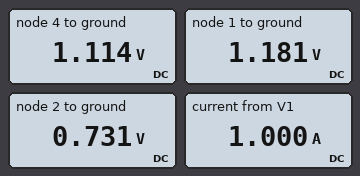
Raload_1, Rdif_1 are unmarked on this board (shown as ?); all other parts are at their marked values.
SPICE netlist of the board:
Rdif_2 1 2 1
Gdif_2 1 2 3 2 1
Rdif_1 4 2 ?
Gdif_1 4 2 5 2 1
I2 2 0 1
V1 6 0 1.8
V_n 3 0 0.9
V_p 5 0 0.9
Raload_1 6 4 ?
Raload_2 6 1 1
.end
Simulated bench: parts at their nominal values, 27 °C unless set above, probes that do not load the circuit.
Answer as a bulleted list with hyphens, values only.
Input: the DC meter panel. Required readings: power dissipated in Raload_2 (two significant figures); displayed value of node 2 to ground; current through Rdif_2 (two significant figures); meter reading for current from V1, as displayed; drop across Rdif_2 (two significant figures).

- 380 mW
- 0.731 V
- 450 mA
- 1.000 A
- 450 mV
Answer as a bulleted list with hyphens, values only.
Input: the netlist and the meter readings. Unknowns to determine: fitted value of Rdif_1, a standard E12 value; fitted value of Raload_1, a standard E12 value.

- 1.8 Ω
- 1.8 Ω
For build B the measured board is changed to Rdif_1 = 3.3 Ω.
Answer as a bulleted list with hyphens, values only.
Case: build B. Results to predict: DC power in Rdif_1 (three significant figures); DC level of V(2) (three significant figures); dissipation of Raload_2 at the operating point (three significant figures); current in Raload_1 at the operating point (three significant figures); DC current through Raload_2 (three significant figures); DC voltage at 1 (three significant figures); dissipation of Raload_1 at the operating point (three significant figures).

- 69.1 mW
- 697 mV
- 426 mW
- 347 mA
- 653 mA
- 1.15 V
- 217 mW
